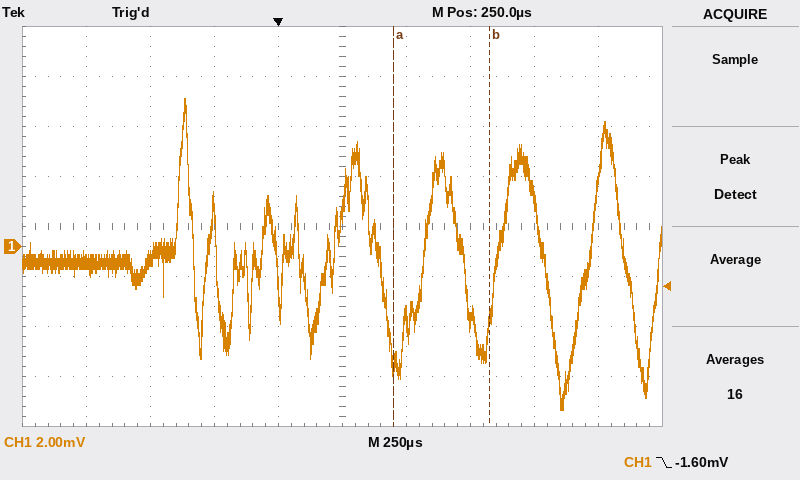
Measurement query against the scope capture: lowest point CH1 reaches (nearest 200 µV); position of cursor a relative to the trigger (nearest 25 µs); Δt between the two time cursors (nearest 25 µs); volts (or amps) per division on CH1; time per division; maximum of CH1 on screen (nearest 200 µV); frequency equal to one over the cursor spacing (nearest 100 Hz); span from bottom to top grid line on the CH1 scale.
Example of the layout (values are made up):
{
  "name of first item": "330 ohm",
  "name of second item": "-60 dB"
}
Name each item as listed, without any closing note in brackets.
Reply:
{
  "lowest point CH1 reaches": "-6.6 mV",
  "position of cursor a relative to the trigger": "+450 µs",
  "Δt between the two time cursors": "375 µs",
  "volts (or amps) per division on CH1": "2 mV",
  "time per division": "250 µs",
  "maximum of CH1 on screen": "6.0 mV",
  "frequency equal to one over the cursor spacing": "2.7 kHz",
  "span from bottom to top grid line on the CH1 scale": "16 mV"
}
